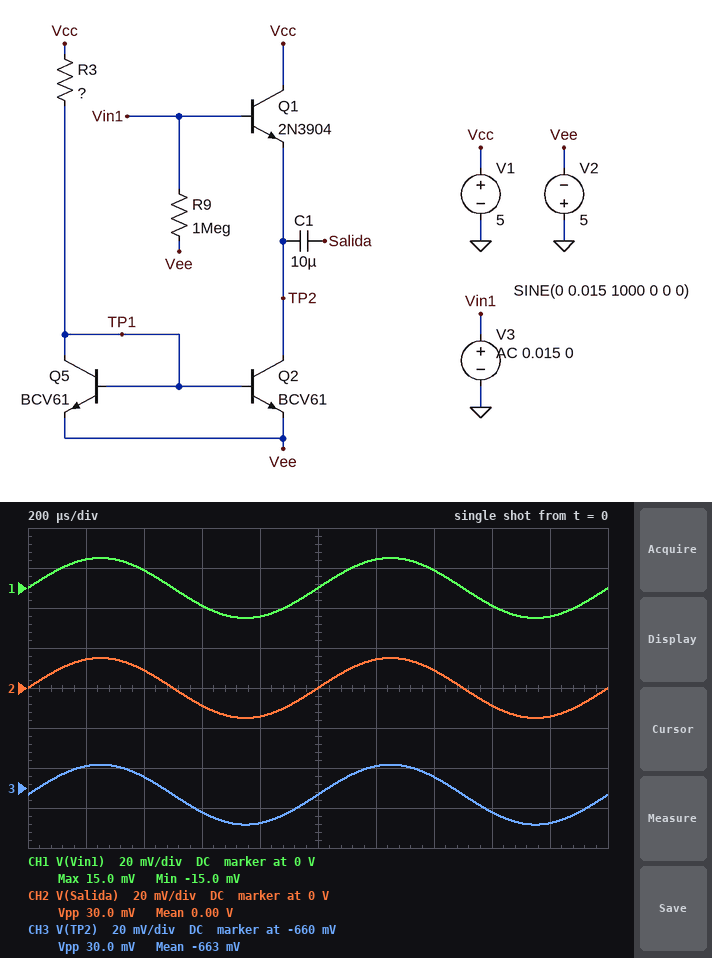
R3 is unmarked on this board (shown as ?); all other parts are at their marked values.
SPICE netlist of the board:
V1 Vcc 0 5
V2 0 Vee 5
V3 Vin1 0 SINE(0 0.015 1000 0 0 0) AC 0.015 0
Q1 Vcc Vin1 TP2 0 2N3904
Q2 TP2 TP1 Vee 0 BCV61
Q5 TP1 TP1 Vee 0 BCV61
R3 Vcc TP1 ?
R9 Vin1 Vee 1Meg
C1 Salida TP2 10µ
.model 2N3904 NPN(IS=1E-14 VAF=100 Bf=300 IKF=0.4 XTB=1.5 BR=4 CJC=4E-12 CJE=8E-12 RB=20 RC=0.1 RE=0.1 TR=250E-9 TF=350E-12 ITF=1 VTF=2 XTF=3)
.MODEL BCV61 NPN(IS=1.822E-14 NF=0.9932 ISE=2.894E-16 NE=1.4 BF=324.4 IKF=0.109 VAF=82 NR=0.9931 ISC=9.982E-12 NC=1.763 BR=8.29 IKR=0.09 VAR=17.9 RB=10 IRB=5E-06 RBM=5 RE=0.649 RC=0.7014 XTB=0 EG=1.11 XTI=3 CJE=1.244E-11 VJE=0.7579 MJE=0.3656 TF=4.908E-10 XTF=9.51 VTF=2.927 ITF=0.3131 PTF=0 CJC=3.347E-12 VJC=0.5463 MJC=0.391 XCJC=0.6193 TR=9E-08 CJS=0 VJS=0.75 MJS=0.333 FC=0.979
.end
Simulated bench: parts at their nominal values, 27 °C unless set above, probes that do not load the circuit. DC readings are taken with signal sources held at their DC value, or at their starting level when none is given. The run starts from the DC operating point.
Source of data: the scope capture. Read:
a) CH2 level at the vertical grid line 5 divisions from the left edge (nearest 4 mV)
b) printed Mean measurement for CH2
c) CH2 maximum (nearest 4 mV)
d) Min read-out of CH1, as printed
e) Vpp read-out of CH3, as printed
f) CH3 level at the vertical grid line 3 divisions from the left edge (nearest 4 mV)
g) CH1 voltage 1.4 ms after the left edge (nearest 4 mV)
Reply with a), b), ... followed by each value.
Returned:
a) 0 V
b) 0.00 V
c) 16 mV
d) -15.0 mV
e) 30.0 mV
f) -672 mV
g) 8 mV
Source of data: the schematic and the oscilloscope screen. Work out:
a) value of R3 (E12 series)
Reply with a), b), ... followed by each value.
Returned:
a) 6.8 kΩ
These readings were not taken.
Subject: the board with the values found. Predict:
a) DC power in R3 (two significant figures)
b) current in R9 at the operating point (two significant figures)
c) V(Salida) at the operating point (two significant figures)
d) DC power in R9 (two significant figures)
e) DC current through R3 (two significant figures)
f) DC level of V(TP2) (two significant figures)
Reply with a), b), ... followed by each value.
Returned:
a) 13 mW
b) 5.0 µA
c) -660 mV
d) 25 µW
e) 1.4 mA
f) -660 mV
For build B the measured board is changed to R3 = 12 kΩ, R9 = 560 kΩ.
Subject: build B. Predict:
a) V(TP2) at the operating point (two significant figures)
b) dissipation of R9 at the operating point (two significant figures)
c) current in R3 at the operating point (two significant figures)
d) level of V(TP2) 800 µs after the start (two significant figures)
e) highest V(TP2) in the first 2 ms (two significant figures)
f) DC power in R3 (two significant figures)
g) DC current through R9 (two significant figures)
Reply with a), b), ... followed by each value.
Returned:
a) -650 mV
b) 45 µW
c) 780 µA
d) -660 mV
e) -630 mV
f) 7.3 mW
g) 8.9 µA
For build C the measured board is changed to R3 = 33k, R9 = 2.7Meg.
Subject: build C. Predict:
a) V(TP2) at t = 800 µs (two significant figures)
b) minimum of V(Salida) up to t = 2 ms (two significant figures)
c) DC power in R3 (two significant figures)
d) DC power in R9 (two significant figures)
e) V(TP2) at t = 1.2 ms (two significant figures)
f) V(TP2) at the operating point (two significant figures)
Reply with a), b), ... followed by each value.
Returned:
a) -640 mV
b) -15 mV
c) 2.7 mW
d) 9.3 µW
e) -610 mV
f) -620 mV
